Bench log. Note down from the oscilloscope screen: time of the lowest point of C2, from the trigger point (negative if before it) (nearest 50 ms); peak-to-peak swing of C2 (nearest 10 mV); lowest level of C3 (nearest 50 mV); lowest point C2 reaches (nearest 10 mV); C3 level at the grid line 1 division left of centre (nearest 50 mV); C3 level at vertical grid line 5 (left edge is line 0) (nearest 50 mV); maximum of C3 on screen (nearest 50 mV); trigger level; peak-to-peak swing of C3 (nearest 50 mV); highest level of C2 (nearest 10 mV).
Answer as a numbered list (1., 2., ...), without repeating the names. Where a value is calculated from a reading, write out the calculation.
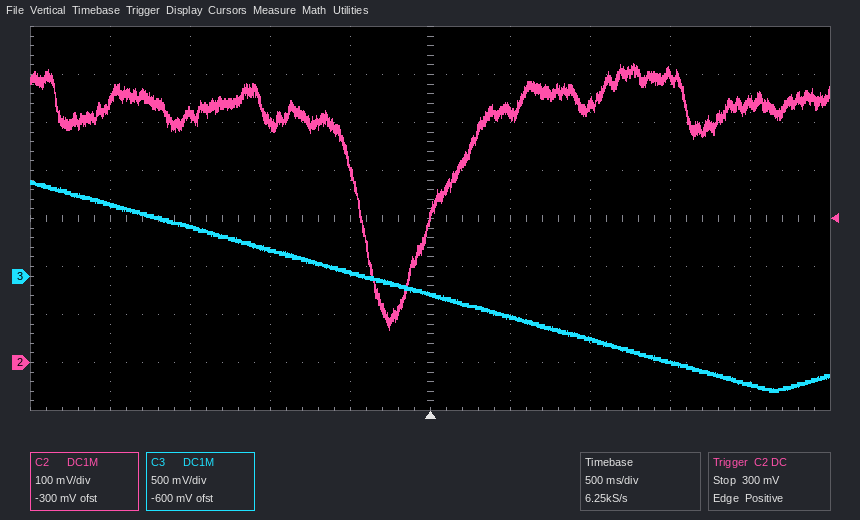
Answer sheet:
1. -250 ms
2. 620 mV − (70 mV) = 550 mV
3. -1.20 V
4. 70 mV
5. 50 mV
6. -200 mV
7. 1.00 V
8. 300 mV
9. 1.00 V − (-1.20 V) = 2.20 V
10. 620 mV
